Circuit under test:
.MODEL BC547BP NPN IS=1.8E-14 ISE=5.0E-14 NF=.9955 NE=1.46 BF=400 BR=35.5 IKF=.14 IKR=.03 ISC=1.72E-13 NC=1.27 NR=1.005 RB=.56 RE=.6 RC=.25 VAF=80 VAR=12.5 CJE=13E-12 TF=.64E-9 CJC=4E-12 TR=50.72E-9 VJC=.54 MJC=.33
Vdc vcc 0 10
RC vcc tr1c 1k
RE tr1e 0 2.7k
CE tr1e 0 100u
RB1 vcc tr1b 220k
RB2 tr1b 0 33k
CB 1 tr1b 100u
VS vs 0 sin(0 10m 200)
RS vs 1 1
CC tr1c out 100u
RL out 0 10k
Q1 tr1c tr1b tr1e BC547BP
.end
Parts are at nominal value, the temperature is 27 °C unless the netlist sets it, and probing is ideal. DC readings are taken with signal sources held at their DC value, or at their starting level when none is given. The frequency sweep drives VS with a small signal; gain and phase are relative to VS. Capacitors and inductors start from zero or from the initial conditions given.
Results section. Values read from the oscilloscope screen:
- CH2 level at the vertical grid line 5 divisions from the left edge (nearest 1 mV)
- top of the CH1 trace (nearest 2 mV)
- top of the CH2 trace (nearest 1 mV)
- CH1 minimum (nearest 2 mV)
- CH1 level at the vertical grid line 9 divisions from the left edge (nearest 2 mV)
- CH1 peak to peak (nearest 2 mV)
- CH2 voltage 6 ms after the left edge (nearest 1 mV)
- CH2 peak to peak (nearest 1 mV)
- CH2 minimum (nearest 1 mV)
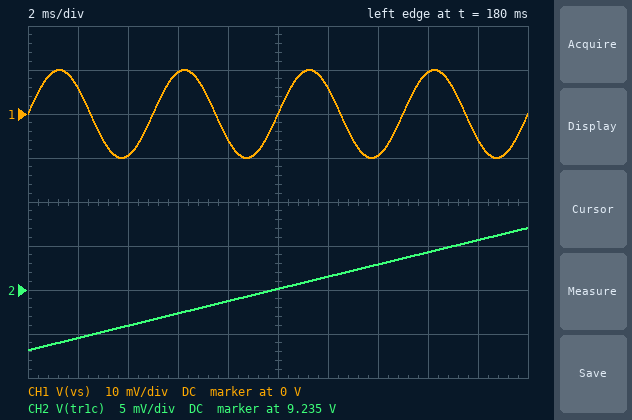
9.235 V
10 mV
9.242 V
-10 mV
-6 mV
20 mV
9.232 V
14 mV
9.228 V
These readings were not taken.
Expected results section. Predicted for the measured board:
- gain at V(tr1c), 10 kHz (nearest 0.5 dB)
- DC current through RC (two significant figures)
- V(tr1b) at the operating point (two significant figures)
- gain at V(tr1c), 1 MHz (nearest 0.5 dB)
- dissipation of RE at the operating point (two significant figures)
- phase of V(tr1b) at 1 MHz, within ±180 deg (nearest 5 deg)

19.0 dB
250 µA
1.3 V
19.0 dB
170 µW
0 deg
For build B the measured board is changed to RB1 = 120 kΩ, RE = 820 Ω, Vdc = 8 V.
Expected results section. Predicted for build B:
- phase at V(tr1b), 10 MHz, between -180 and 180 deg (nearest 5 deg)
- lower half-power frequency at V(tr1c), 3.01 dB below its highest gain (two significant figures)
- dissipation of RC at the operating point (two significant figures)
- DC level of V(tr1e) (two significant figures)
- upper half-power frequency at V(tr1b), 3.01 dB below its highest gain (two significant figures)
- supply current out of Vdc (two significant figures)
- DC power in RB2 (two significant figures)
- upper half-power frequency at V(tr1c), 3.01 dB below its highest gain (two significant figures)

0 deg
72 Hz
1.4 mW
980 mV
2.3 GHz
1.2 mA
79 µW
90 MHz
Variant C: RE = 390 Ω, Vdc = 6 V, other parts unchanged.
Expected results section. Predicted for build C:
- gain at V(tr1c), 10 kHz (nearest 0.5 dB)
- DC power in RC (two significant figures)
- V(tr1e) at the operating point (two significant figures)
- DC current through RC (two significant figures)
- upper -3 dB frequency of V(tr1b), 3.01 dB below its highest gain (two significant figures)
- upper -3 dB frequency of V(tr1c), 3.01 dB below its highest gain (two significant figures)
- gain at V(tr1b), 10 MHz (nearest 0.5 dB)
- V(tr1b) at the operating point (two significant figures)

21.5 dB
120 µW
130 mV
340 µA
4.0 GHz
93 MHz
0 dB
740 mV
